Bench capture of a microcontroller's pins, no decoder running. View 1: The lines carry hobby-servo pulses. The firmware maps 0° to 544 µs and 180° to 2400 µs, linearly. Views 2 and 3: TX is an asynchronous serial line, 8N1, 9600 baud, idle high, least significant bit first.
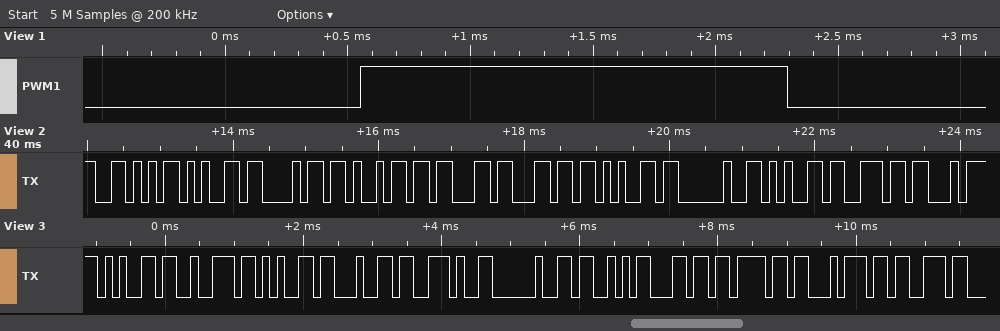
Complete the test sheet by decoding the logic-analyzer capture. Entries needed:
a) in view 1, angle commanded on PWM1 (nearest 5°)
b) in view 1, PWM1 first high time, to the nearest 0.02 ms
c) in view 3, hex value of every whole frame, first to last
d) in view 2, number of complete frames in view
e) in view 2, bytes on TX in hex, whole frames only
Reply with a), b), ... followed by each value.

a) 115°
b) 1.74 ms
c) 65 72 65 64 2E 20 53 6C 6F 74 73
d) 10
e) 56 65 68 69 63 6C 65 20 65 6E
